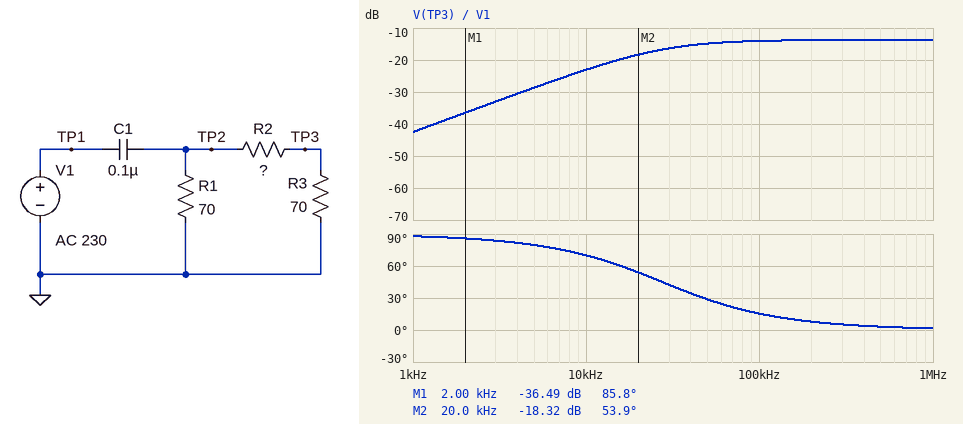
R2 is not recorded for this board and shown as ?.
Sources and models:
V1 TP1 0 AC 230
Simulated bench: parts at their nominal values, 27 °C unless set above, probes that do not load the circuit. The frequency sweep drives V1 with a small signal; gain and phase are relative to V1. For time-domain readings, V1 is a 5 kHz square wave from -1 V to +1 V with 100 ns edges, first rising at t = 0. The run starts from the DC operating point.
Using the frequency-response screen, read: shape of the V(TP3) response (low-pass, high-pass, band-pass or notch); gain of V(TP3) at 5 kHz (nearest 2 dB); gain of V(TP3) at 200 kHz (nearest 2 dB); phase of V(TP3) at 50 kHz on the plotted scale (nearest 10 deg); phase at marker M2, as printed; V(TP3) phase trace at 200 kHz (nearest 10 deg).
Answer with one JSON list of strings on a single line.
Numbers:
["high-pass", "-28 dB", "-14 dB", "30 deg", "53.9 deg", "10 deg"]
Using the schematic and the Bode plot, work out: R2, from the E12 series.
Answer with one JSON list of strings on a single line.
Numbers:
["270 Ω"]
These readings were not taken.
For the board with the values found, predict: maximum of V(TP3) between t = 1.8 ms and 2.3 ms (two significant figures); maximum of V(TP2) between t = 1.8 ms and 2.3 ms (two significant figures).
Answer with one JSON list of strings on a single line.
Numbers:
["410 mV", "2.0 V"]
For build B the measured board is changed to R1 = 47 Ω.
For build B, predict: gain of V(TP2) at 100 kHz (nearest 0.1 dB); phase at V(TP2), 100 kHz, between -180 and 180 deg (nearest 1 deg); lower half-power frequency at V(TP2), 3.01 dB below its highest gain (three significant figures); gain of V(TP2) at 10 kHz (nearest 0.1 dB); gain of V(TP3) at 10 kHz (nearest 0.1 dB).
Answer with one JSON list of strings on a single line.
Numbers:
["-0.6 dB", "21 deg", "38.5 kHz", "-12.0 dB", "-25.7 dB"]
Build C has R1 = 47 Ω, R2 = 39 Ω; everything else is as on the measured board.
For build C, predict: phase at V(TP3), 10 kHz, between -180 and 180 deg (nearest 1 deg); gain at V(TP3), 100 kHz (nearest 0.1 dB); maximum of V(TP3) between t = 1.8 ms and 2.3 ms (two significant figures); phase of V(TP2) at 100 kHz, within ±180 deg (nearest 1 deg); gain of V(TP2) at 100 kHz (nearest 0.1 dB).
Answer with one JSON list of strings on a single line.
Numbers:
["78 deg", "-4.8 dB", "1.3 V", "26 deg", "-0.9 dB"]
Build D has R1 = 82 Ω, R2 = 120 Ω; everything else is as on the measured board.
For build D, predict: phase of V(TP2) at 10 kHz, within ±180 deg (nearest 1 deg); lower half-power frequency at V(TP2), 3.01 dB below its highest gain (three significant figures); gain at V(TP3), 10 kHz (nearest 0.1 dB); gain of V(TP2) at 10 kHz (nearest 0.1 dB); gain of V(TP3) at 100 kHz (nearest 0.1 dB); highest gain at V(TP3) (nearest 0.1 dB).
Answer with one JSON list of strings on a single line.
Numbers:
["70 deg", "27.8 kHz", "-18.1 dB", "-9.4 dB", "-9.0 dB", "-8.7 dB"]
